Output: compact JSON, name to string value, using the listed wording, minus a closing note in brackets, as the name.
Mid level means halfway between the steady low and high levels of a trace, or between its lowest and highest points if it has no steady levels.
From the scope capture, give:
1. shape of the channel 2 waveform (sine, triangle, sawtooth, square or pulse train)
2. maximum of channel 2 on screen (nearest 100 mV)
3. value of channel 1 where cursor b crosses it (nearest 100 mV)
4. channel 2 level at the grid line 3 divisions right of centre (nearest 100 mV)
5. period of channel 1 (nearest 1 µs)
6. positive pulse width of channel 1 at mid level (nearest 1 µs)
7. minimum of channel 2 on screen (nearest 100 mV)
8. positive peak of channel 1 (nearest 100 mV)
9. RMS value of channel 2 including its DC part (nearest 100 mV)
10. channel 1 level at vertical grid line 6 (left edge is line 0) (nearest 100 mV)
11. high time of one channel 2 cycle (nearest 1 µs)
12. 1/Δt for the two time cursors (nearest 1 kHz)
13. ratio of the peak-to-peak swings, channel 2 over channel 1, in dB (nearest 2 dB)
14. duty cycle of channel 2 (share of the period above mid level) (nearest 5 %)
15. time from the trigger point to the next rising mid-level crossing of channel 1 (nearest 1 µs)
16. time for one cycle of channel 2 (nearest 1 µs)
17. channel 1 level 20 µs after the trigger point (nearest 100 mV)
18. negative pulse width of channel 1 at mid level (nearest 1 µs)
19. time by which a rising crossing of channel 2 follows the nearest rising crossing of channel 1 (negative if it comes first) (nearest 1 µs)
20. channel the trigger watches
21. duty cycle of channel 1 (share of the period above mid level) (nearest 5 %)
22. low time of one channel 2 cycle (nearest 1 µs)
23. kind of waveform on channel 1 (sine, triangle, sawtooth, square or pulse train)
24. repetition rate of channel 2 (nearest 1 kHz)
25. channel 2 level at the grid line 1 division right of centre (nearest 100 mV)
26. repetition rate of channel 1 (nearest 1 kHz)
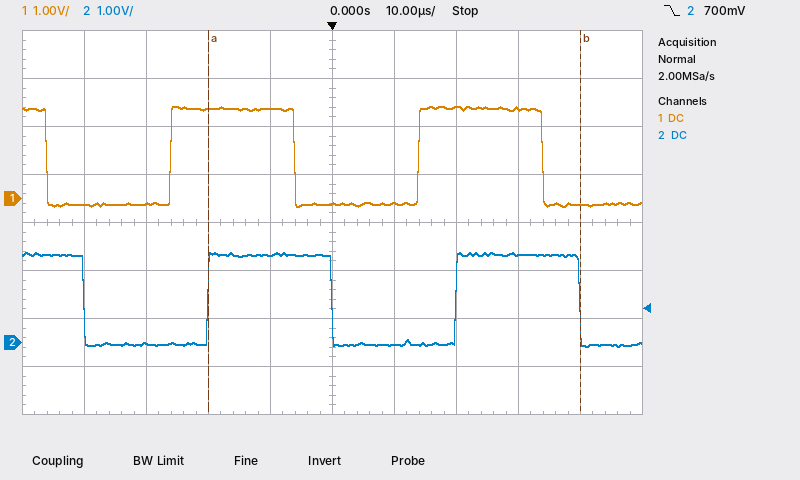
{"shape of the channel 2 waveform": "square", "maximum of channel 2 on screen": "1.9 V", "value of channel 1 where cursor b crosses it": "-100 mV", "channel 2 level at the grid line 3 divisions right of centre": "1.8 V", "period of channel 1": "40 µs", "positive pulse width of channel 1 at mid level": "20 µs", "minimum of channel 2 on screen": "-100 mV", "positive peak of channel 1": "1.9 V", "RMS value of channel 2 including its DC part": "1.3 V", "channel 1 level at vertical grid line 6 (left edge is line 0)": "-100 mV", "high time of one channel 2 cycle": "20 µs", "1/Δt for the two time cursors": "17 kHz", "ratio of the peak-to-peak swings, channel 2 over channel 1, in dB": "0 dB", "duty cycle of channel 2 (share of the period above mid level)": "50 %", "time from the trigger point to the next rising mid-level crossing of channel 1": "14 µs", "time for one cycle of channel 2": "40 µs", "channel 1 level 20 µs after the trigger point": "1.9 V", "negative pulse width of channel 1 at mid level": "20 µs", "time by which a rising crossing of channel 2 follows the nearest rising crossing of channel 1 (negative if it comes first)": "+6 µs", "channel the trigger watches": "channel 2", "duty cycle of channel 1 (share of the period above mid level)": "50 %", "low time of one channel 2 cycle": "20 µs", "kind of waveform on channel 1": "square", "repetition rate of channel 2": "25 kHz", "channel 2 level at the grid line 1 division right of centre": "0.0 V", "repetition rate of channel 1": "25 kHz"}
